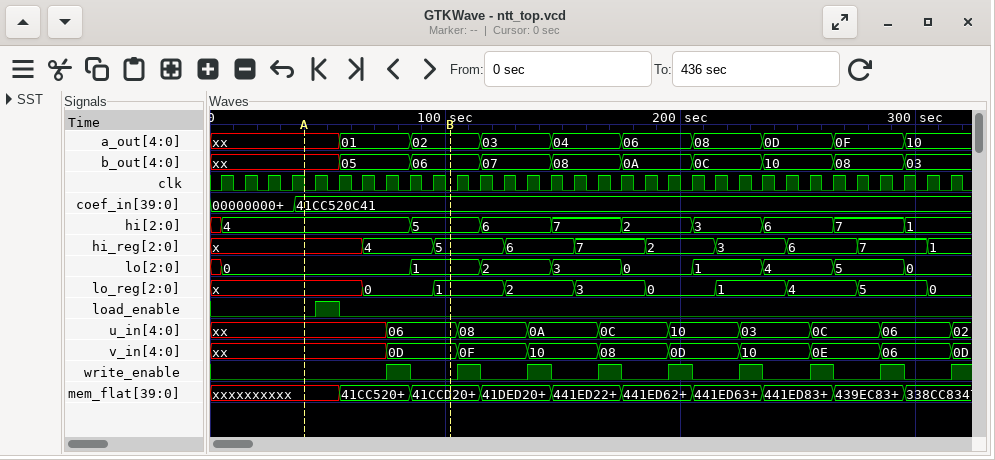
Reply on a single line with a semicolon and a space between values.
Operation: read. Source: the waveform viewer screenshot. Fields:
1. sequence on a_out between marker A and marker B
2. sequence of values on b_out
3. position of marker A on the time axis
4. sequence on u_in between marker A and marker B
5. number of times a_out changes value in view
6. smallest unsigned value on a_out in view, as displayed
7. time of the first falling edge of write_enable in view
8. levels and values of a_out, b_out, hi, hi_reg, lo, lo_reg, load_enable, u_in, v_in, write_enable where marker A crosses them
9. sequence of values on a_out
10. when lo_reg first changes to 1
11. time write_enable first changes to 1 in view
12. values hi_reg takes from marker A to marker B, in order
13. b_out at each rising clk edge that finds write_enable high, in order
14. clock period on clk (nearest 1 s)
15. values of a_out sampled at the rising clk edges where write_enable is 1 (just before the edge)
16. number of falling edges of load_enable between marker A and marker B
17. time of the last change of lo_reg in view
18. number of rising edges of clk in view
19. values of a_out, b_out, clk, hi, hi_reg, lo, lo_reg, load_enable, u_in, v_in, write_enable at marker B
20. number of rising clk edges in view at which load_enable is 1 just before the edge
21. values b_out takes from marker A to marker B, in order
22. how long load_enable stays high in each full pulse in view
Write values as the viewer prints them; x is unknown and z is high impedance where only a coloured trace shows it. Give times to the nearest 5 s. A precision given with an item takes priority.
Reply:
xx, 01, 02; xx, 05, 06, 07, 08, 0A, 0C, 10, 08, 03; 40 s; xx, 06; 9; 01; 85 s; a_out=xx, b_out=xx, hi=4, hi_reg=x, lo=0, lo_reg=x, load_enable=0, u_in=xx, v_in=xx, write_enable=0; xx, 01, 02, 03, 04, 06, 08, 0D, 0F, 10; 95 s; 75 s; x, 4, 5; 05, 06, 07, 08, 0A, 0C, 10, 08; 10 s; 01, 02, 03, 04, 06, 08, 0D, 0F; 1; 305 s; 32; a_out=02, b_out=06, clk=0, hi=5, hi_reg=5, lo=1, lo_reg=1, load_enable=0, u_in=06, v_in=0D, write_enable=0; 1; xx, 05, 06; 10 s
